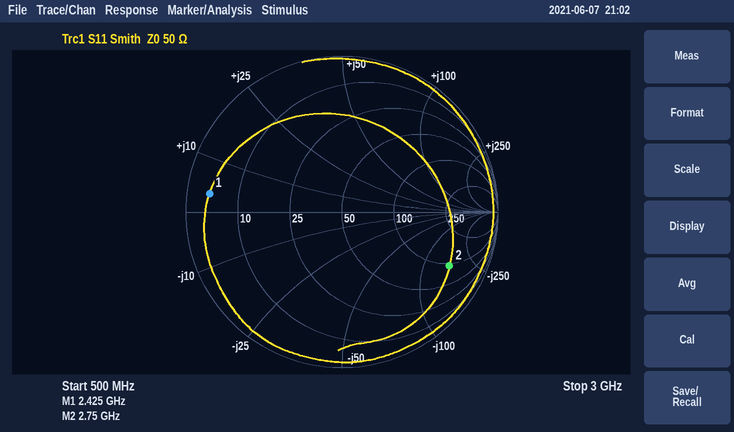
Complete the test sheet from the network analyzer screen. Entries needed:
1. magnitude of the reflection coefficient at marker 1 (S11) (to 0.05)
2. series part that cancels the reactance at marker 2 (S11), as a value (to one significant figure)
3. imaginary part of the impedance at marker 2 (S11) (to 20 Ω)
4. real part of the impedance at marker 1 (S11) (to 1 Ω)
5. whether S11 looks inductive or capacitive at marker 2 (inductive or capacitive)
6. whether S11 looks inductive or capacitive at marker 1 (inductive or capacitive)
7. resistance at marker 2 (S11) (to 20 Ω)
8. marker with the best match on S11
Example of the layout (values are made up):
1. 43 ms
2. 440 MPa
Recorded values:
1. 0.85
2. 9 nH
3. -160 Ω
4. 4 Ω
5. capacitive
6. inductive
7. 100 Ω
8. marker 2
